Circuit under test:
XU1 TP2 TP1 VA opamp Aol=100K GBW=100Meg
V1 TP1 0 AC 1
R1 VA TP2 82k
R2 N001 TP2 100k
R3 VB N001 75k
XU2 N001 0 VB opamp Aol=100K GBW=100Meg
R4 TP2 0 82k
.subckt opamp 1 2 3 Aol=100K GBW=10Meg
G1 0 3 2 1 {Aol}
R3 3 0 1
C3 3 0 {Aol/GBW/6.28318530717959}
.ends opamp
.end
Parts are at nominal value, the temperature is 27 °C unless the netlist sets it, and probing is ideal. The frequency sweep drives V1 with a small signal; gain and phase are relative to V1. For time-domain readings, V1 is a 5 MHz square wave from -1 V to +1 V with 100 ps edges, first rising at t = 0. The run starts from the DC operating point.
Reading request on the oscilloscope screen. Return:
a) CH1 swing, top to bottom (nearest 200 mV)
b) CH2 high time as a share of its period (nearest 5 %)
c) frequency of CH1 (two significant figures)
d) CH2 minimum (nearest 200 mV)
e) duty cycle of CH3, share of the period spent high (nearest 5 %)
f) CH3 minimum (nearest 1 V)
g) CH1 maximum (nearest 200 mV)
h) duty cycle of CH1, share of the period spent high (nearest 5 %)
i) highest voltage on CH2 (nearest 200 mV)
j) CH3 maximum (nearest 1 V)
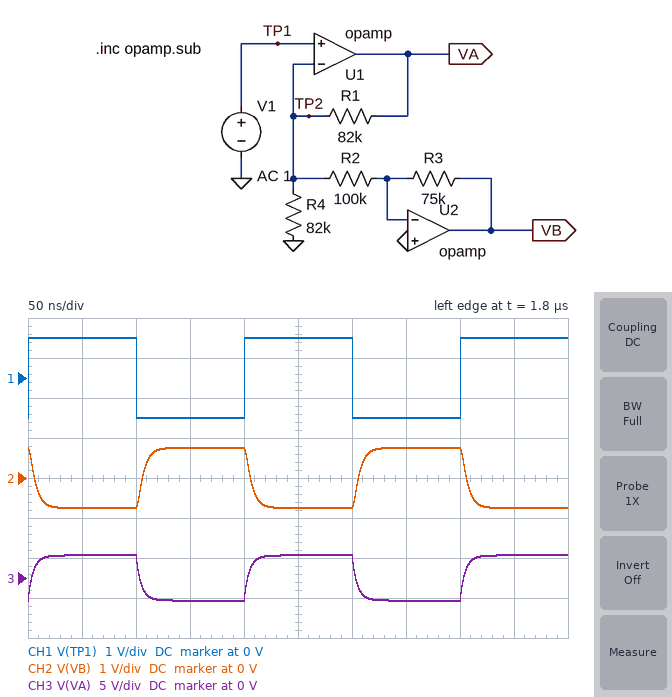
2.0 V
50 %
5.0 MHz
-800 mV
50 %
-3 V
1.0 V
50 %
800 mV
3 V
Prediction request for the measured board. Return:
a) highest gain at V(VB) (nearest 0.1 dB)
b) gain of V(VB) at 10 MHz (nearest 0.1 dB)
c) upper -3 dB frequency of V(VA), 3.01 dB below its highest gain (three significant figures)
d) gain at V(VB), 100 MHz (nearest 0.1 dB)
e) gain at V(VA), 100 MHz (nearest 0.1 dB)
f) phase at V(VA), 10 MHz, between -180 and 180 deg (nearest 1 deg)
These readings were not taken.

-2.5 dB
-3.0 dB
32.4 MHz
-17.5 dB
-0.8 dB
-17 deg
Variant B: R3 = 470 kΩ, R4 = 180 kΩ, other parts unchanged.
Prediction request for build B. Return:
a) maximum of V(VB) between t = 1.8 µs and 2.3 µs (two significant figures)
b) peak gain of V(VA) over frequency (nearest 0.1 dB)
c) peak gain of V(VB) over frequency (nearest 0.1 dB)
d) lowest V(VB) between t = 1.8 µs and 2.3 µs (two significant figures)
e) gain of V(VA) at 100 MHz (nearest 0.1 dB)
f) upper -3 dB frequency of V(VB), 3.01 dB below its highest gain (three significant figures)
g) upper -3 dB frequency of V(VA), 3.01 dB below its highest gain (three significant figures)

4.7 V
7.1 dB
13.4 dB
-4.7 V
-1.7 dB
14.6 MHz
23.6 MHz
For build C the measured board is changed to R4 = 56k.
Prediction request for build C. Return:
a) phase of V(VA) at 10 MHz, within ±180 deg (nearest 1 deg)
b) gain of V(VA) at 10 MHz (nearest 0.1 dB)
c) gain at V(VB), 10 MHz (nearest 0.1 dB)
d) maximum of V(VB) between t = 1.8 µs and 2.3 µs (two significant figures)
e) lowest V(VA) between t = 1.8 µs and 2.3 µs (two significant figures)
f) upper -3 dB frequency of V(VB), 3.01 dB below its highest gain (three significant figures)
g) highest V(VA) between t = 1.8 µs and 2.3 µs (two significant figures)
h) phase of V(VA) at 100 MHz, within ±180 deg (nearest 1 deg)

-19 deg
9.8 dB
-3.1 dB
750 mV
-3.3 V
24.5 MHz
3.3 V
-72 deg
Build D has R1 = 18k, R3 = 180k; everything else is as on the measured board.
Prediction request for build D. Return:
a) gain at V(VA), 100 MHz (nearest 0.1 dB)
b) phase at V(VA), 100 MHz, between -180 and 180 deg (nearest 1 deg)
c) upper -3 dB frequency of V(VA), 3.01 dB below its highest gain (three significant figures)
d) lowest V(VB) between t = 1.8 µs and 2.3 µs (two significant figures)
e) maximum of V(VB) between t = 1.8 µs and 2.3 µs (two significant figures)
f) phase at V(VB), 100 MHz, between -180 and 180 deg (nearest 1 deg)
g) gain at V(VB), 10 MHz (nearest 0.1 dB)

-2.1 dB
-53 deg
63.6 MHz
-1.8 V
1.8 V
58 deg
4.7 dB
